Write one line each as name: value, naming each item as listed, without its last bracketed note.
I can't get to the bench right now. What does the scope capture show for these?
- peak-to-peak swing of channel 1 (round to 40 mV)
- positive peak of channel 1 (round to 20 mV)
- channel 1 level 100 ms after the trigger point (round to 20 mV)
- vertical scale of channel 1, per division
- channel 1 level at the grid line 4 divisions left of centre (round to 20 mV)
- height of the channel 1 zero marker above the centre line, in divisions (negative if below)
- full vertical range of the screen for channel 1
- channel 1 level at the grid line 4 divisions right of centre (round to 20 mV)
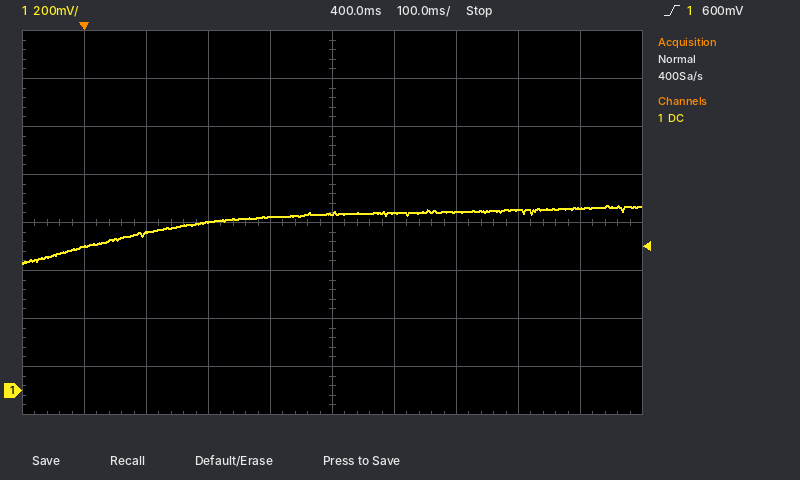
peak-to-peak swing of channel 1: 240 mV
positive peak of channel 1: 780 mV
channel 1 level 100 ms after the trigger point: 660 mV
vertical scale of channel 1, per division: 200 mV
channel 1 level at the grid line 4 divisions left of centre: 600 mV
height of the channel 1 zero marker above the centre line, in divisions: -3.5 div
full vertical range of the screen for channel 1: 1.6 V
channel 1 level at the grid line 4 divisions right of centre: 760 mV
